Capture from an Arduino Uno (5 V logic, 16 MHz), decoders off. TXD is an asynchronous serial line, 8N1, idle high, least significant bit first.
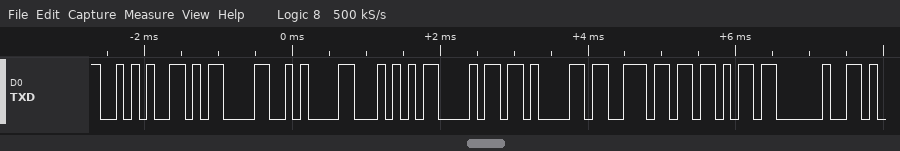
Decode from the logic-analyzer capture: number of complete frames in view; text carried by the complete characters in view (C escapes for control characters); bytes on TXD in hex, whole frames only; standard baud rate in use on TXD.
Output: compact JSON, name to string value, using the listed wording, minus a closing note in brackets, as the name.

{"number of complete frames in view": "9", "text carried by the complete characters in view": "\"*\\r\\nThank \"", "bytes on TXD in hex, whole frames only": "0x2A 0x0D 0x0A 0x54 0x68 0x61 0x6E 0x6B 0x20", "standard baud rate in use on TXD": "9600 baud"}
